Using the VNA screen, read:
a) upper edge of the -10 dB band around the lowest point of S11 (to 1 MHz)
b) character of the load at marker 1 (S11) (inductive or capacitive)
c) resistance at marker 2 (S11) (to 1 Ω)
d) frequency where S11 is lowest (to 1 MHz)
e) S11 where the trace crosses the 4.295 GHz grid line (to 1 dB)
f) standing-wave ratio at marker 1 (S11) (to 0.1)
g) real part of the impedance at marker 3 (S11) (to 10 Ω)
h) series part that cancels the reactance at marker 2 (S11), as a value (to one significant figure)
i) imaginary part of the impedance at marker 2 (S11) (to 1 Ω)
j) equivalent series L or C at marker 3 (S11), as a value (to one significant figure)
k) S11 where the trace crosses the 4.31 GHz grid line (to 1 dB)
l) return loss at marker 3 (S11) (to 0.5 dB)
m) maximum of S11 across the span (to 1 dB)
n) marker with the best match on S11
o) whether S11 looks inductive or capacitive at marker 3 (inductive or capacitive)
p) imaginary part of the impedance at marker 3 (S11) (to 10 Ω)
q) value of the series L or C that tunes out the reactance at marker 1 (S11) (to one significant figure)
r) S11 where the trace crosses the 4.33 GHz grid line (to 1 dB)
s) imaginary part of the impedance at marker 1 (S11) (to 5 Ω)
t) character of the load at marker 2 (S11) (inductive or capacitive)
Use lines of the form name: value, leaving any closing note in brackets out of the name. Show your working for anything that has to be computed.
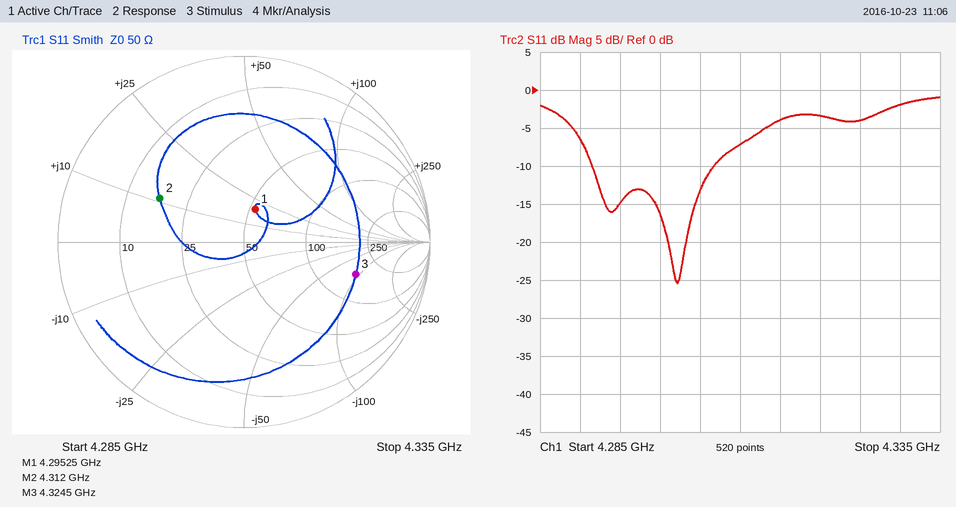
upper edge of the -10 dB band around the lowest point of S11: 4.307 GHz
character of the load at marker 1 (S11): inductive
resistance at marker 2 (S11): 17 Ω
frequency where S11 is lowest: 4.302 GHz
S11 where the trace crosses the 4.295 GHz grid line: -15 dB
standing-wave ratio at marker 1 (S11): 1.5
real part of the impedance at marker 3 (S11): 160 Ω
series part that cancels the reactance at marker 2 (S11), as a value: C = 1/(2π × 4.312 GHz × 11 Ω) ≈ 3 pF
imaginary part of the impedance at marker 2 (S11): +11 Ω
equivalent series L or C at marker 3 (S11), as a value: C = 1/(2π × 4.3245 GHz × 90 Ω) ≈ 409 fF, so 400 fF to one significant figure
S11 where the trace crosses the 4.31 GHz grid line: -7 dB
return loss at marker 3 (S11): 4.0 dB
maximum of S11 across the span: -1 dB
marker with the best match on S11: marker 1
whether S11 looks inductive or capacitive at marker 3: capacitive
imaginary part of the impedance at marker 3 (S11): -90 Ω
value of the series L or C that tunes out the reactance at marker 1 (S11): C = 1/(2π × 4.29525 GHz × 20 Ω) ≈ 2 pF
S11 where the trace crosses the 4.33 GHz grid line: -2 dB
imaginary part of the impedance at marker 1 (S11): +20 Ω
character of the load at marker 2 (S11): inductive
